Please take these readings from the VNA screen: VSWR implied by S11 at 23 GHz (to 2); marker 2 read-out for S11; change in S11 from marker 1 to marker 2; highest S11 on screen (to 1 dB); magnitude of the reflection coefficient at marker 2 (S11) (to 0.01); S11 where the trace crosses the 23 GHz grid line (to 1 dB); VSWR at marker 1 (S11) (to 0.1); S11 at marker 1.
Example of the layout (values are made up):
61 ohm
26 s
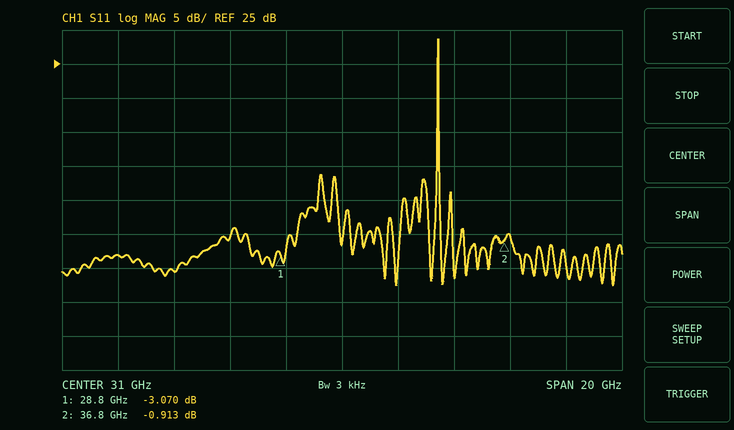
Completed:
6
-0.913 dB
2.157 dB
29 dB
0.90
-3 dB
5.7
-3.070 dB
